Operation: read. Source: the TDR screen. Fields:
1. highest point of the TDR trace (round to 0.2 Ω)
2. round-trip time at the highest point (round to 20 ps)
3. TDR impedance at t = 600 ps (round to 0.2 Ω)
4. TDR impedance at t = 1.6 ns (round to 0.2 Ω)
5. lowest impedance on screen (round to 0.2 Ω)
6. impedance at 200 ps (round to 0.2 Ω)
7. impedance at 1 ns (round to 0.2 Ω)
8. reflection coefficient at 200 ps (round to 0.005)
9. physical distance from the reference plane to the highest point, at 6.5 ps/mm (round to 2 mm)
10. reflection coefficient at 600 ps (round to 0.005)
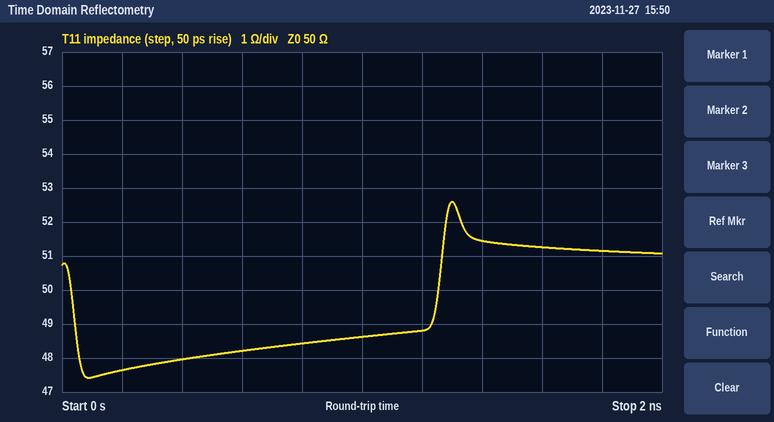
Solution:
52.6 Ω
1.30 ns
48.2 Ω
51.2 Ω
47.4 Ω
47.6 Ω
48.6 Ω
-0.025
100 mm
-0.020
